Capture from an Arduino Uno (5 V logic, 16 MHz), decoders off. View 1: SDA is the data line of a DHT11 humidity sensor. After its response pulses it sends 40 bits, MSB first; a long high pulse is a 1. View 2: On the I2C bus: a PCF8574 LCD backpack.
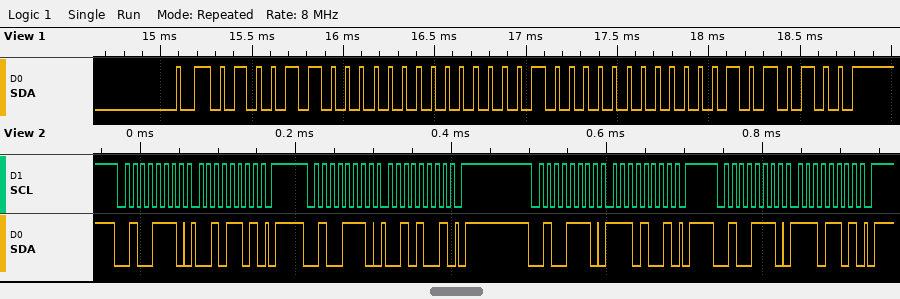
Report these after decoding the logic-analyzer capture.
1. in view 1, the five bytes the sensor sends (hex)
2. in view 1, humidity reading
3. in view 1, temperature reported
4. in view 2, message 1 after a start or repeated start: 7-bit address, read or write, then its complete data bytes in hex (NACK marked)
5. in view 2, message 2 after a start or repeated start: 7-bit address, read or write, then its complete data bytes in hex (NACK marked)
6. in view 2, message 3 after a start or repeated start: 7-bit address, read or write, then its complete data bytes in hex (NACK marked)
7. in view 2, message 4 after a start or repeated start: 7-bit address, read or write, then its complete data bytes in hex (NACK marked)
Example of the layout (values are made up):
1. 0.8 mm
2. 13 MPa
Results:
1. 4C 00 08 00 54
2. 76 %
3. 8.0 °C
4. 0x27 write: 2D
5. 0x27 write: 29
6. 0x27 write: E9
7. 0x27 write: ED
